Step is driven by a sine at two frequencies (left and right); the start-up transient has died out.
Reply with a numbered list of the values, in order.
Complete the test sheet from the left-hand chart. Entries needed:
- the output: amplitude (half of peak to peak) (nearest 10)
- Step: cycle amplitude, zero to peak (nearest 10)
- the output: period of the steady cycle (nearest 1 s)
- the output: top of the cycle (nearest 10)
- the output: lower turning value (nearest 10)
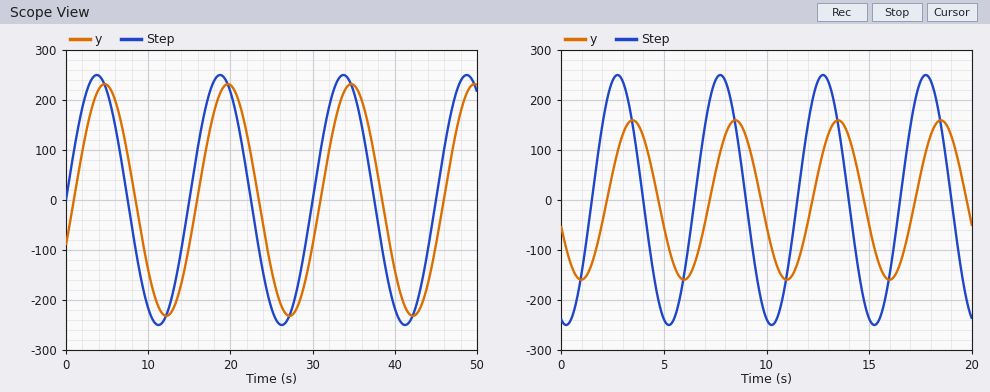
1. 230
2. 250
3. 15 s
4. 230
5. -230
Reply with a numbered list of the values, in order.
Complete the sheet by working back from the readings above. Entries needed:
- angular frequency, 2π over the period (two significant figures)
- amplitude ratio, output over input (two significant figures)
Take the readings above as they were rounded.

1. 0.42 rad/s
2. 0.92
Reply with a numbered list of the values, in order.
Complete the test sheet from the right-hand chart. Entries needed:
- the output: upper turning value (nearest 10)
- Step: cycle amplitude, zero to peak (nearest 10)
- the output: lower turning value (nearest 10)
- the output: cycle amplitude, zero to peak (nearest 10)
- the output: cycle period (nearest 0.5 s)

1. 160
2. 250
3. -160
4. 160
5. 5.0 s
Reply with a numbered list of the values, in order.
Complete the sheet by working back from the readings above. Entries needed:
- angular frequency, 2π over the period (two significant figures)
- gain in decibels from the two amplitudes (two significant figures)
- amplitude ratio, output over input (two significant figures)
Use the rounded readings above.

1. 1.3 rad/s
2. -3.9 dB
3. 0.64
